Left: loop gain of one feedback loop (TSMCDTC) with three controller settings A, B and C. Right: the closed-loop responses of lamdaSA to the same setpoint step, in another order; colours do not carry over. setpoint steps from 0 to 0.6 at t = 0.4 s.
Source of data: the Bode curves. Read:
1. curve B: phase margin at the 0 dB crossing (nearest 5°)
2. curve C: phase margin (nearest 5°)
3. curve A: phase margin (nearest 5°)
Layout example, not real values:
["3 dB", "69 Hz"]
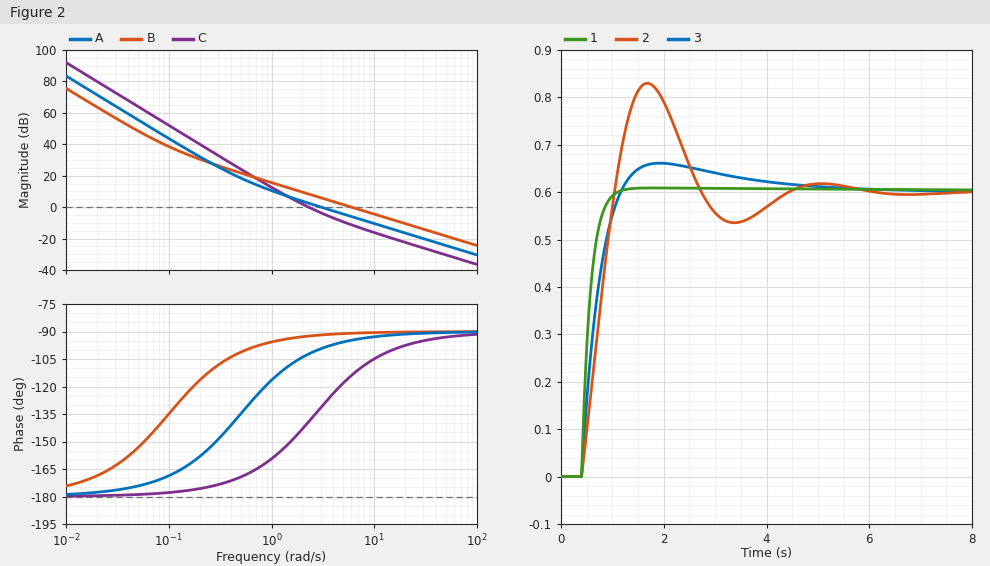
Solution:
["90°", "40°", "80°"]
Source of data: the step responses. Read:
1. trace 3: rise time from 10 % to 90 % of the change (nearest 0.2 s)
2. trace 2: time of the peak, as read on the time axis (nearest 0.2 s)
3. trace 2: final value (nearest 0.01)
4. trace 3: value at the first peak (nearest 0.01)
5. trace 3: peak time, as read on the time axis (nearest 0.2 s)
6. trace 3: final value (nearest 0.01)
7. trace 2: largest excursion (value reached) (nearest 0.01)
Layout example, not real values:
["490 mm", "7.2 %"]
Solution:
["0.6 s", "1.6 s", "0.60", "0.66", "2.0 s", "0.60", "0.83"]
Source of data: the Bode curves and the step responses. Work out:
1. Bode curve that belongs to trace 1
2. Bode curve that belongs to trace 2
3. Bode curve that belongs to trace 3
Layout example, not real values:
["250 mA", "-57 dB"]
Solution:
["B", "C", "A"]
